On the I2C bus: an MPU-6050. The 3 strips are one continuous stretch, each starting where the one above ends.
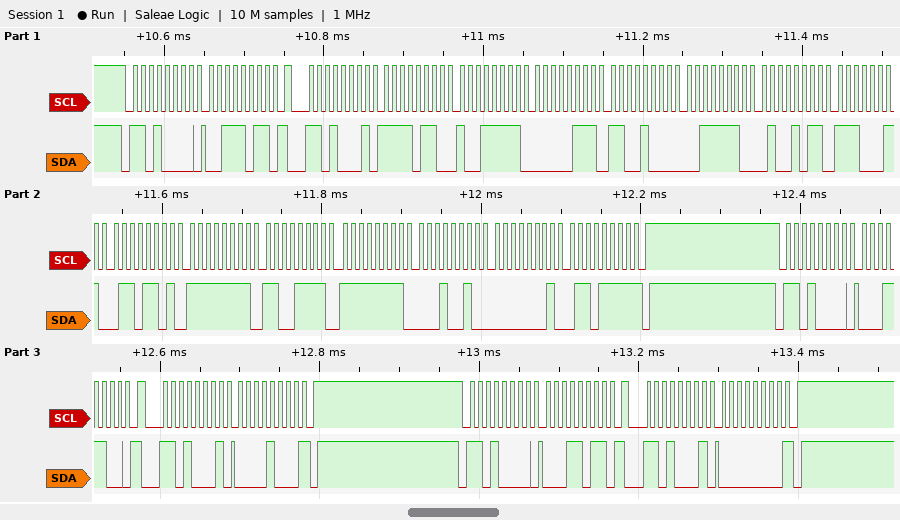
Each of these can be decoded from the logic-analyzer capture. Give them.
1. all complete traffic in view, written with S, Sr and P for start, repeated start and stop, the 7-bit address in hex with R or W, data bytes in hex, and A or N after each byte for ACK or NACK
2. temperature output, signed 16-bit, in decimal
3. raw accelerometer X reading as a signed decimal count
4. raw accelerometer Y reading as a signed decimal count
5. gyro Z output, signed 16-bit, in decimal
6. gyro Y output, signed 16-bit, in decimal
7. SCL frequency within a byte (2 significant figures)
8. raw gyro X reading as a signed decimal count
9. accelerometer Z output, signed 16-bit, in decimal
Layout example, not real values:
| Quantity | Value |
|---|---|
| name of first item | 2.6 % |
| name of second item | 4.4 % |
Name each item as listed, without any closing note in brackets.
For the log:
| Quantity | Value |
|---|---|
| all complete traffic in view, written with S, Sr and P for start, repeated start and stop, the 7-bit address in hex with R or W, data bytes in hex, and A or N after each byte for ACK or NACK | S 68W A 3B A Sr 68R A F6 A 9F A 07 A C8 A 3E A 4B A E3 A 6D A FF A CF A FF A 12 A 01 A 6F N P S 68W A 1C A Sr 68R A 08 N P S 68W A 1B A Sr 68R A 00 N P |
| temperature output, signed 16-bit, in decimal | -7315 |
| raw accelerometer X reading as a signed decimal count | -2401 |
| raw accelerometer Y reading as a signed decimal count | 1992 |
| gyro Z output, signed 16-bit, in decimal | 367 |
| gyro Y output, signed 16-bit, in decimal | -238 |
| SCL frequency within a byte | 100 kHz |
| raw gyro X reading as a signed decimal count | -49 |
| accelerometer Z output, signed 16-bit, in decimal | 15947 |
